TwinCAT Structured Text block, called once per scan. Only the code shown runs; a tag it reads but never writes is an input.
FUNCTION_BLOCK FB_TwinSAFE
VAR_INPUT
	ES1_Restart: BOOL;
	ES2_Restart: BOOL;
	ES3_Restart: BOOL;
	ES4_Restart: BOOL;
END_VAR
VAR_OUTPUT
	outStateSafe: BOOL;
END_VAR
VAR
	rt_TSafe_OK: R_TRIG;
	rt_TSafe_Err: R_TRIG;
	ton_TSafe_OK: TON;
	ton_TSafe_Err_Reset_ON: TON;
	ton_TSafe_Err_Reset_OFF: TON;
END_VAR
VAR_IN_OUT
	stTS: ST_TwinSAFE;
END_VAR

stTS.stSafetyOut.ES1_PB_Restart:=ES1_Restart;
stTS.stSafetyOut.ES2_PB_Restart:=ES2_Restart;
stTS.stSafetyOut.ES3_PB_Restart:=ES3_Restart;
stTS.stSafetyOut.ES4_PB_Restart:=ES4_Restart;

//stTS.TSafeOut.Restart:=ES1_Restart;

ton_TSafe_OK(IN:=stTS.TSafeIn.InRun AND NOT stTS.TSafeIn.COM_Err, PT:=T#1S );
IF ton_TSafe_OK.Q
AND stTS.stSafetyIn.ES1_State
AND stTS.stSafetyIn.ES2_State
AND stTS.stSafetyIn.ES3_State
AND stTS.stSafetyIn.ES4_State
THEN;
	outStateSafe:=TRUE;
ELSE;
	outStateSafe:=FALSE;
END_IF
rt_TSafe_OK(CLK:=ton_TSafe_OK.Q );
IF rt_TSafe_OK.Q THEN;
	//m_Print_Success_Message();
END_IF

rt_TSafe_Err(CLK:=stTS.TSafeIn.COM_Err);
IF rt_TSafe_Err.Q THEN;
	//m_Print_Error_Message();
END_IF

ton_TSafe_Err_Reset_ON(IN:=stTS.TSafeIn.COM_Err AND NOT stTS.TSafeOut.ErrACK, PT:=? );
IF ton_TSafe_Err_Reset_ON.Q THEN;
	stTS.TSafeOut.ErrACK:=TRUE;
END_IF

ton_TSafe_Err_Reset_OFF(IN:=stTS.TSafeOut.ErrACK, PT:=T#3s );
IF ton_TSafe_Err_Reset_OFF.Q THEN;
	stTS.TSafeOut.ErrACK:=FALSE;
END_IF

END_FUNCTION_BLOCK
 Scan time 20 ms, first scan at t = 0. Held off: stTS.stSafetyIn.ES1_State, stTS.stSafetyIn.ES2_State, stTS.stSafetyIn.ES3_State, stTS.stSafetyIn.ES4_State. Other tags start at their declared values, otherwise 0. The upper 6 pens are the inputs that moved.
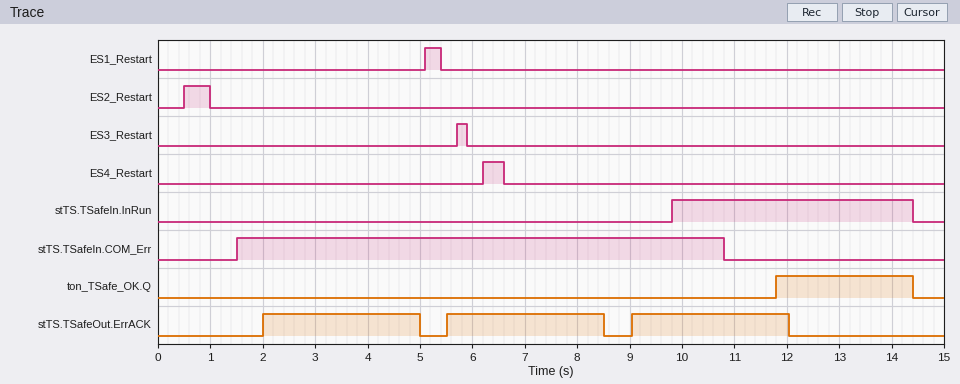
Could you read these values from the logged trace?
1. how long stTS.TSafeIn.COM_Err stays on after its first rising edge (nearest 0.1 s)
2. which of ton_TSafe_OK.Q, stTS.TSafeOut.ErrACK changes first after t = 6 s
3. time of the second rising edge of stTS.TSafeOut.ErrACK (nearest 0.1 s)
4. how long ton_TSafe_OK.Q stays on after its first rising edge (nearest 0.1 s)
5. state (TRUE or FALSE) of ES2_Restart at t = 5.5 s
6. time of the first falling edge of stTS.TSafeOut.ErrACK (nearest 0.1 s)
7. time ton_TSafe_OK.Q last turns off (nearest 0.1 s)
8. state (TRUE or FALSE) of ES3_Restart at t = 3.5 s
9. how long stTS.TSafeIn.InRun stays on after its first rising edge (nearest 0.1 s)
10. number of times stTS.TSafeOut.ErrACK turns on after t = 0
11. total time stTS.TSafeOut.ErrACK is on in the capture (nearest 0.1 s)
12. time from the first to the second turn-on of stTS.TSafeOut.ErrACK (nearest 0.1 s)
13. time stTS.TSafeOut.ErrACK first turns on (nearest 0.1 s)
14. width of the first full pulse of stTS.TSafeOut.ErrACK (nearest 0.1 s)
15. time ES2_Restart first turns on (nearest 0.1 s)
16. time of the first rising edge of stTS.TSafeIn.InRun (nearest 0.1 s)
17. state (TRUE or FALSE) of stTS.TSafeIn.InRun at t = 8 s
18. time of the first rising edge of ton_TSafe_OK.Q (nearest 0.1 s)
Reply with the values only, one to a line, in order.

9.3 s
stTS.TSafeOut.ErrACK
5.5 s
2.6 s
FALSE
5.0 s
14.4 s
FALSE
4.6 s
3
9.0 s
3.5 s
2.0 s
3.0 s
0.5 s
9.8 s
FALSE
11.8 s
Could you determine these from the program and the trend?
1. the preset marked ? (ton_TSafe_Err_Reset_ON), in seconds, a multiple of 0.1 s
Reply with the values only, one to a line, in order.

0.5 s
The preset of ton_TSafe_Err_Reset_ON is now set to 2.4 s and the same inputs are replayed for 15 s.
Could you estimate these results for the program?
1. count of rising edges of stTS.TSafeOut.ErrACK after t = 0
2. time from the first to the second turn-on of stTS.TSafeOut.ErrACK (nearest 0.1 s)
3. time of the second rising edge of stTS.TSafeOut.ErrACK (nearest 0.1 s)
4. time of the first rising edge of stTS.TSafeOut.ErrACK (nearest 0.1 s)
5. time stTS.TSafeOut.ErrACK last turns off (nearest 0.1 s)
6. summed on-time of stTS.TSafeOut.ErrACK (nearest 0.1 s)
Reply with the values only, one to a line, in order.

2
5.4 s
9.3 s
3.9 s
12.3 s
6.0 s
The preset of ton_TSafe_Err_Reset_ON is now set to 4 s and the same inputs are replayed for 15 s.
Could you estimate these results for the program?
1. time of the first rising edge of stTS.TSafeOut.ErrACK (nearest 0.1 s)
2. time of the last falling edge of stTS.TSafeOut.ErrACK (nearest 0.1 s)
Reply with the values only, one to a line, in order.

5.5 s
8.5 s
